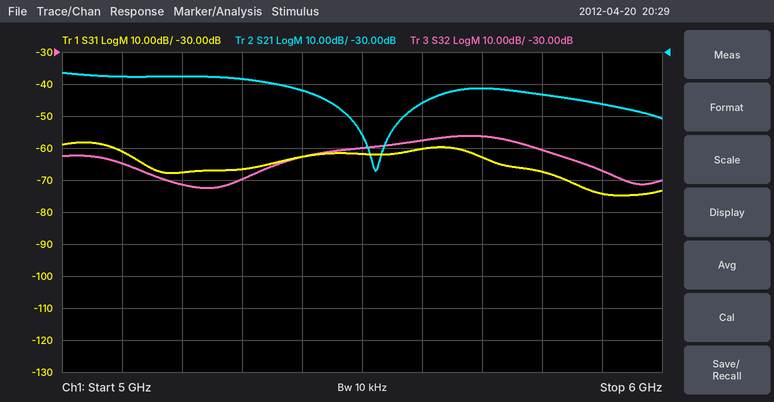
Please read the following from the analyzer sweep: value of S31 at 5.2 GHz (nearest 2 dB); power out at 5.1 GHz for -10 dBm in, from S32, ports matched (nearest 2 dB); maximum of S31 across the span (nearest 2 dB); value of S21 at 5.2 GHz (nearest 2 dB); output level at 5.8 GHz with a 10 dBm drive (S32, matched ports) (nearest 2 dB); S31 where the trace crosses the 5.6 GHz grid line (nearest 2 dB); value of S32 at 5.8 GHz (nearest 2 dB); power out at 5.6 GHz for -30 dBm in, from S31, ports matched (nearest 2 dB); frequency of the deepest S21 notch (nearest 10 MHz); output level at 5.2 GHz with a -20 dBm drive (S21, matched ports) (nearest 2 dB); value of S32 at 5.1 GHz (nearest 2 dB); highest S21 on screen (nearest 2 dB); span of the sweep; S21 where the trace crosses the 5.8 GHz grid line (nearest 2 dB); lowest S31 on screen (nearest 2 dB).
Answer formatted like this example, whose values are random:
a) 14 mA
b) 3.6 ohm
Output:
a) -68 dB
b) -74 dBm
c) -58 dB
d) -38 dB
e) -50 dBm
f) -60 dB
g) -60 dB
h) -90 dBm
i) 5.52 GHz
j) -58 dBm
k) -64 dB
l) -36 dB
m) 1 GHz
n) -44 dB
o) -74 dB
